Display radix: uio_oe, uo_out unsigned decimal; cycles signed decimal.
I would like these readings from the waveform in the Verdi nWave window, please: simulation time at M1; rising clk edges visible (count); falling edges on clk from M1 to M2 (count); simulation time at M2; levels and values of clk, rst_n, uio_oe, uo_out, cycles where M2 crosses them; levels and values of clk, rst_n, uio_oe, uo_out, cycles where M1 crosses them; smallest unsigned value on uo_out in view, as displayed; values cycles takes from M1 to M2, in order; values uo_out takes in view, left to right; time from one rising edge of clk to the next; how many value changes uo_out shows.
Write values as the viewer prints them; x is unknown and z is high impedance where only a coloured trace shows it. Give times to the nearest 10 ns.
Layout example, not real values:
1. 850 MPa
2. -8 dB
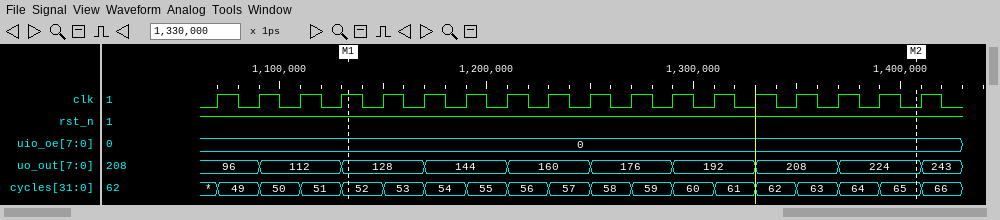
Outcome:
1. 1130 ns
2. 18
3. 14
4. 1410 ns
5. clk=0, rst_n=1, uio_oe=0, uo_out=224, cycles=65
6. clk=1, rst_n=1, uio_oe=0, uo_out=128, cycles=52
7. 96
8. 52, 53, 54, 55, 56, 57, 58, 59, 60, 61, 62, 63, 64, 65
9. 96, 112, 128, 144, 160, 176, 192, 208, 224, 243
10. 20 ns
11. 9
